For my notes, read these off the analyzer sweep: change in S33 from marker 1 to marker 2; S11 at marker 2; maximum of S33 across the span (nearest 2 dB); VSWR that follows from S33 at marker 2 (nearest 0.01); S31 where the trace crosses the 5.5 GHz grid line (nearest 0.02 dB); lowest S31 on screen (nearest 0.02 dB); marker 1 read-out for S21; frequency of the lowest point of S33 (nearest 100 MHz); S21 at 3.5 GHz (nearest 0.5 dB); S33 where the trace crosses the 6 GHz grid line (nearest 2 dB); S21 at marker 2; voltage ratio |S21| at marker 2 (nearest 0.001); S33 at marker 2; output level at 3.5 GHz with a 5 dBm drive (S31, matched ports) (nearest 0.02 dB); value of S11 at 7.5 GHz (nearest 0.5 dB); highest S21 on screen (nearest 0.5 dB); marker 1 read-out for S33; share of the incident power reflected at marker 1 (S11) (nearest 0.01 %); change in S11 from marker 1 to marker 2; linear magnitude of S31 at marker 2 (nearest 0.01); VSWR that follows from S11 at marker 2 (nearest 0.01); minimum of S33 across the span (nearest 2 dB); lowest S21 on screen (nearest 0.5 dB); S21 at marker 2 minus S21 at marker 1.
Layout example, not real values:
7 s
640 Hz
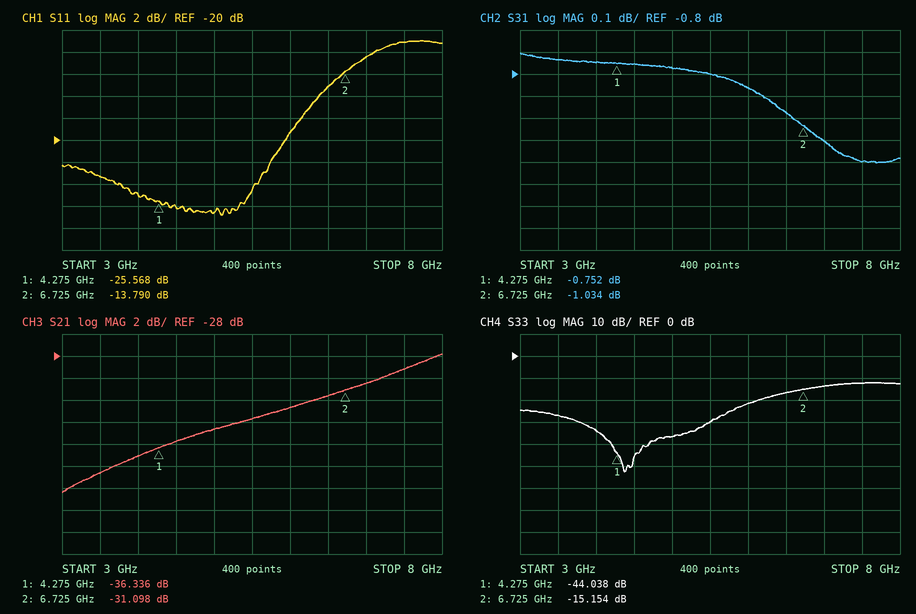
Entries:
28.884 dB
-13.790 dB
-12 dB
1.42
-0.80 dB
-1.20 dB
-36.336 dB
4.4 GHz
-38.5 dB
-22 dB
-31.098 dB
0.028
-15.154 dB
4.26 dBm
-11.0 dB
-28.0 dB
-44.038 dB
0.28 %
11.778 dB
0.89
1.51
-52 dB
-40.5 dB
5.238 dB
